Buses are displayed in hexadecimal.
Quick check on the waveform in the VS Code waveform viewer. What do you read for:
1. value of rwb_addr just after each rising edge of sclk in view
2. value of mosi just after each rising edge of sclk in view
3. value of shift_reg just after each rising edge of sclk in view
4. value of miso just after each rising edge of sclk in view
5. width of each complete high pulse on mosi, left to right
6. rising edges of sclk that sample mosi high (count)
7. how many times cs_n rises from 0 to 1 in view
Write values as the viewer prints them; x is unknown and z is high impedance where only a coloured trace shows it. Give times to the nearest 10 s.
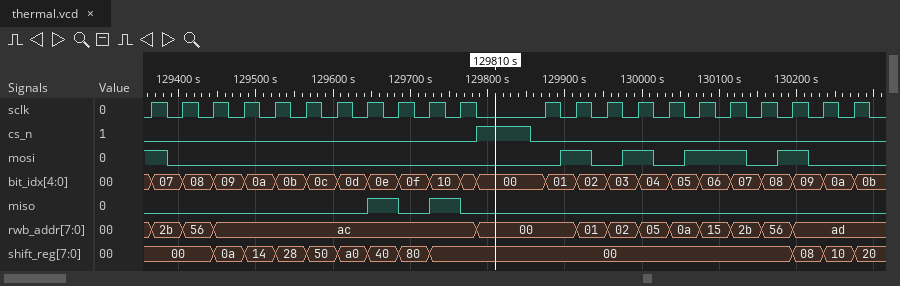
2b, 56, ac, ac, ac, ac, ac, ac, ac, ac, ac, 00, 01, 02, 05, 0a, 15, 2b, 56, ad, ad, ad
1 0 0 0 0 0 0 0 0 0 0 0 1 0 1 0 1 1 0 1 0 0
00, 00, 0a, 14, 28, 50, a0, 40, 80, 00, 00, 00, 00, 00, 00, 00, 00, 00, 00, 08, 10, 20
0 0 0 0 0 0 0 1 0 1 0 0 0 0 0 0 0 0 0 0 0 0
40 s, 40 s, 80 s, 40 s
6
1
